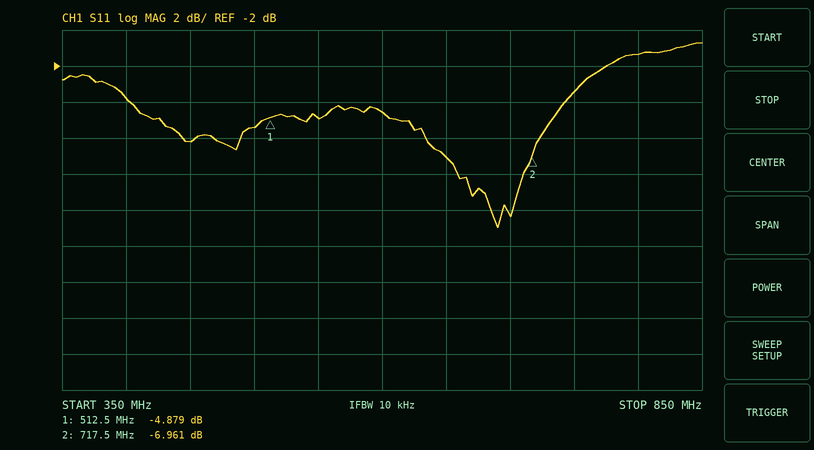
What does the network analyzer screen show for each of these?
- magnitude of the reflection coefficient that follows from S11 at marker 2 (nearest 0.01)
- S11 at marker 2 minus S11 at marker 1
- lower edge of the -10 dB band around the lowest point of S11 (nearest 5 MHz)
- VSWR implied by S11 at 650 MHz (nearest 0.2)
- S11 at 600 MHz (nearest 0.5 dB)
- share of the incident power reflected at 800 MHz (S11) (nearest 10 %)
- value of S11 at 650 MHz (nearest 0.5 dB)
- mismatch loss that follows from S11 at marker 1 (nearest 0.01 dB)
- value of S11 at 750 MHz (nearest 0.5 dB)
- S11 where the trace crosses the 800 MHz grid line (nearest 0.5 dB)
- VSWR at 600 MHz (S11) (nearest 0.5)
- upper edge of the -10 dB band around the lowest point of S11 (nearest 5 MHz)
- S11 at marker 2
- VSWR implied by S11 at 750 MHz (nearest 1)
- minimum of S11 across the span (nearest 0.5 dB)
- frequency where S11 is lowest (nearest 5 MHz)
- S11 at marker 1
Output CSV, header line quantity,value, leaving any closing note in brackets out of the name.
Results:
quantity,value
magnitude of the reflection coefficient that follows from S11 at marker 2,0.45
S11 at marker 2 minus S11 at marker 1,-2.082 dB
lower edge of the -10 dB band around the lowest point of S11,685 MHz
VSWR implied by S11 at 650 MHz,2.6
S11 at 600 MHz,-4.5 dB
share of the incident power reflected at 800 MHz (S11),70 %
value of S11 at 650 MHz,-7.0 dB
mismatch loss that follows from S11 at marker 1,1.71 dB
value of S11 at 750 MHz,-3.5 dB
S11 where the trace crosses the 800 MHz grid line,-1.5 dB
VSWR at 600 MHz (S11),4.0
upper edge of the -10 dB band around the lowest point of S11,695 MHz
S11 at marker 2,-6.961 dB
VSWR implied by S11 at 750 MHz,5
minimum of S11 across the span,-11.0 dB
frequency where S11 is lowest,690 MHz
S11 at marker 1,-4.879 dB
